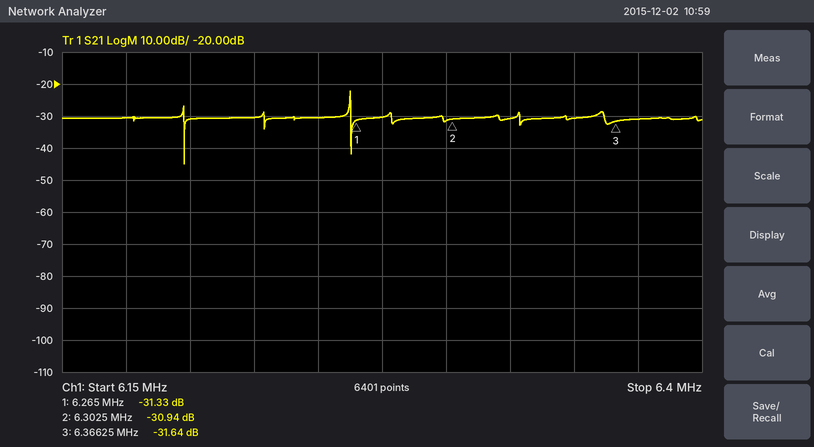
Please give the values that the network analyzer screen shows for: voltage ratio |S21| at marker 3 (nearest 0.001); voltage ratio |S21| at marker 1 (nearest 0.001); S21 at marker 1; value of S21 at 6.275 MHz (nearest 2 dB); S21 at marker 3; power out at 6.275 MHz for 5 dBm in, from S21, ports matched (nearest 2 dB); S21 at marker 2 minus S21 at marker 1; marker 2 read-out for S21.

0.026
0.027
-31.33 dB
-30 dB
-31.64 dB
-26 dBm
0.39 dB
-30.94 dB
